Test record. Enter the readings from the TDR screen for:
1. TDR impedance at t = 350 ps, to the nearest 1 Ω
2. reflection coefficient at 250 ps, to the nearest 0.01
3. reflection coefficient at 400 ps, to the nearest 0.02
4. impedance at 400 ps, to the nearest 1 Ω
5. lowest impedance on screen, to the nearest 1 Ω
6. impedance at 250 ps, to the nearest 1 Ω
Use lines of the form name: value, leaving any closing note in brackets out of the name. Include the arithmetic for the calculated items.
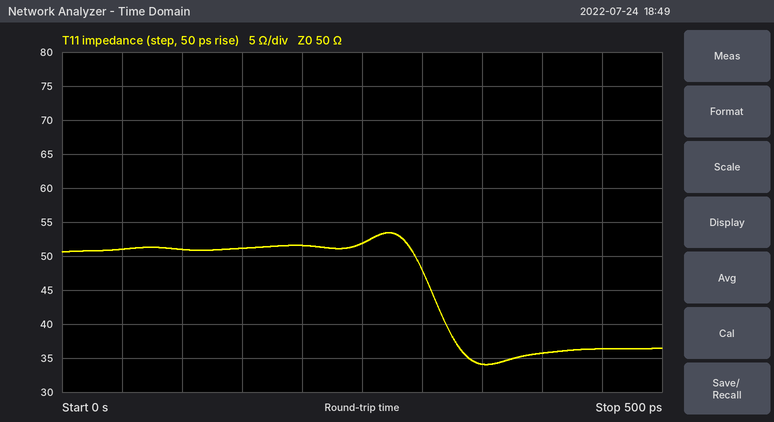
TDR impedance at t = 350 ps, to the nearest 1 Ω: 34 Ω
reflection coefficient at 250 ps, to the nearest 0.01: (52 − 50)/(52 + 50) ≈ +0.02
reflection coefficient at 400 ps, to the nearest 0.02: (36 − 50)/(36 + 50) ≈ -0.16
impedance at 400 ps, to the nearest 1 Ω: 36 Ω
lowest impedance on screen, to the nearest 1 Ω: 34 Ω
impedance at 250 ps, to the nearest 1 Ω: 52 Ω
